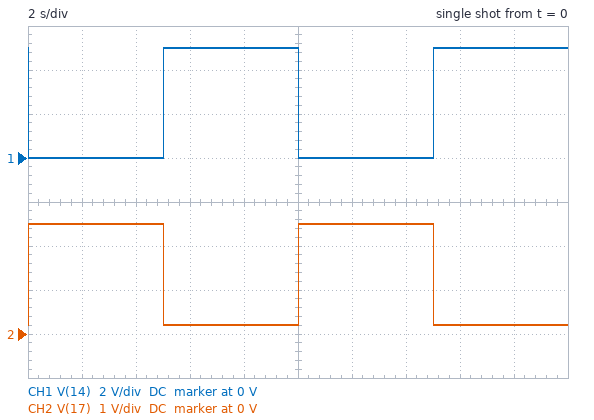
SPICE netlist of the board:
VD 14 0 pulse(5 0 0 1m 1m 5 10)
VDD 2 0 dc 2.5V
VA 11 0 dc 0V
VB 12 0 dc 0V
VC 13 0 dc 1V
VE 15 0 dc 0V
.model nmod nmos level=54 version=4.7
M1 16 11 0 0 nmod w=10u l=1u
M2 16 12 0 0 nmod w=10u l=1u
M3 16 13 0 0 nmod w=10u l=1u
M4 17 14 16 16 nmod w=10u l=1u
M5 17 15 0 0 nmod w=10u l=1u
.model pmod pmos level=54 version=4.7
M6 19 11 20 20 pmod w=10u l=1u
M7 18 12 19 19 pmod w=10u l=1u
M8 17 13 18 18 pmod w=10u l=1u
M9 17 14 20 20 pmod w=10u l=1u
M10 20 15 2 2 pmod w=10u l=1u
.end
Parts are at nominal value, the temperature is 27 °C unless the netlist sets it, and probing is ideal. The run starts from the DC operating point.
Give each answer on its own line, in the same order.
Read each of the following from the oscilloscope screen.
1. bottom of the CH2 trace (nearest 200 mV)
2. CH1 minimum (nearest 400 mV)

200 mV
0 V
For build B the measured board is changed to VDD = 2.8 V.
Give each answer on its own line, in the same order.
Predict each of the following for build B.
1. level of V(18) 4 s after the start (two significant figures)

2.8 V
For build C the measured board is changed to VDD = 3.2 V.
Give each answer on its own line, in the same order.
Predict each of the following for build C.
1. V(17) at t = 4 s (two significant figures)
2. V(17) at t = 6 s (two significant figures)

3.2 V
440 mV
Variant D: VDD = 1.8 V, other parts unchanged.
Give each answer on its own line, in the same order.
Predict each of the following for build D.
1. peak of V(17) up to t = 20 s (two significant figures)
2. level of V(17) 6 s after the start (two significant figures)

1.8 V
59 mV
